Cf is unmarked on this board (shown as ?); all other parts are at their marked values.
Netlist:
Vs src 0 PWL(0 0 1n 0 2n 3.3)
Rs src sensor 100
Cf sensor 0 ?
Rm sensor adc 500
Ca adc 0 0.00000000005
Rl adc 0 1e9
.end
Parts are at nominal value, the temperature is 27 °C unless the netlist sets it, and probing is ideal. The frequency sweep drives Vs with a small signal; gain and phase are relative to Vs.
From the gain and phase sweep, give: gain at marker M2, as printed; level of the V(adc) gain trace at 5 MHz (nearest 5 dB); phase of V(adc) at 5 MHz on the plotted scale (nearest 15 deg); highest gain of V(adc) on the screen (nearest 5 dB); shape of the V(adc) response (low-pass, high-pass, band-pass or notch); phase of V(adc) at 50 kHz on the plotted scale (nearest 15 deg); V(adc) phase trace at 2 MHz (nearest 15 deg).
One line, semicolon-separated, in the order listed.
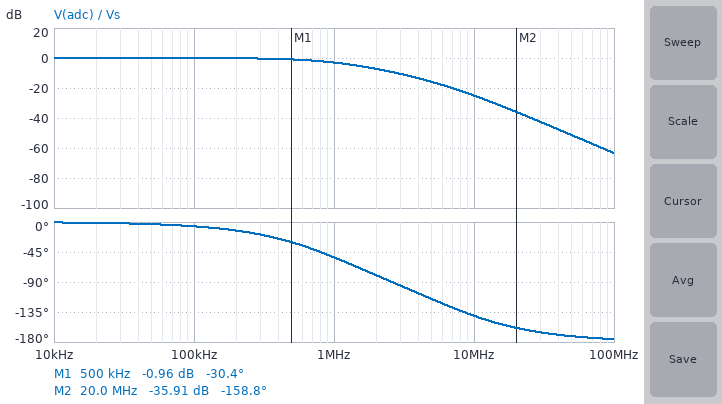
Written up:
-35.91 dB; -15 dB; -120 deg; 0 dB; low-pass; 0 deg; -75 deg
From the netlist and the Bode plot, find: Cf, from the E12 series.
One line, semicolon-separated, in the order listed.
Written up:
1.5 nF
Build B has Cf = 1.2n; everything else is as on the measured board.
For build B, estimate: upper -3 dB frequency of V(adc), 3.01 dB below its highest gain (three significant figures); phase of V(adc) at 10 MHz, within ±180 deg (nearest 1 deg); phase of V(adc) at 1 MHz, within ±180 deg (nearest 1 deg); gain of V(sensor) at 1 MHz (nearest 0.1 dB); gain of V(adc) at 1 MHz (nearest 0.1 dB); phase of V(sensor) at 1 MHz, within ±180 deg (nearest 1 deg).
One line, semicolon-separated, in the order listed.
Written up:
1.22 MHz; -139 deg; -47 deg; -2.1 dB; -2.2 dB; -38 deg
